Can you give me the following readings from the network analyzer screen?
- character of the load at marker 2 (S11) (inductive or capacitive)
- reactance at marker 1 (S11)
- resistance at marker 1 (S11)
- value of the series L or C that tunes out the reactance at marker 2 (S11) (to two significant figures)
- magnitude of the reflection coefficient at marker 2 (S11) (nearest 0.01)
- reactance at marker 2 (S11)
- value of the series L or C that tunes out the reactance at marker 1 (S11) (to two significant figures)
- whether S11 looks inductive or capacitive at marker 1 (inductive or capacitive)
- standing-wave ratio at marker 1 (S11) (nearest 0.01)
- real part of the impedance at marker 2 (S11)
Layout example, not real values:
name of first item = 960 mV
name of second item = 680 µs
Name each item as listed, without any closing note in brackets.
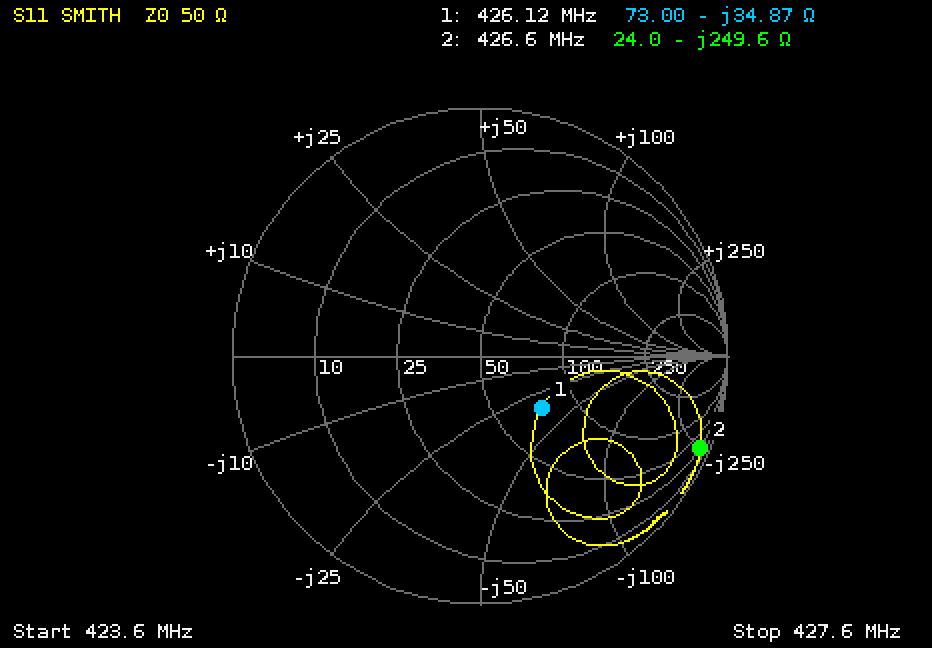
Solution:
character of the load at marker 2 (S11) = capacitive
reactance at marker 1 = -34.87 Ω
resistance at marker 1 = 73.00 Ω
value of the series L or C that tunes out the reactance at marker 2 (S11) = 93 nH
magnitude of the reflection coefficient at marker 2 (S11) = 0.96
reactance at marker 2 = -249.6 Ω
value of the series L or C that tunes out the reactance at marker 1 (S11) = 13 nH
whether S11 looks inductive or capacitive at marker 1 = capacitive
standing-wave ratio at marker 1 (S11) = 1.97
real part of the impedance at marker 2 = 24.0 Ω
